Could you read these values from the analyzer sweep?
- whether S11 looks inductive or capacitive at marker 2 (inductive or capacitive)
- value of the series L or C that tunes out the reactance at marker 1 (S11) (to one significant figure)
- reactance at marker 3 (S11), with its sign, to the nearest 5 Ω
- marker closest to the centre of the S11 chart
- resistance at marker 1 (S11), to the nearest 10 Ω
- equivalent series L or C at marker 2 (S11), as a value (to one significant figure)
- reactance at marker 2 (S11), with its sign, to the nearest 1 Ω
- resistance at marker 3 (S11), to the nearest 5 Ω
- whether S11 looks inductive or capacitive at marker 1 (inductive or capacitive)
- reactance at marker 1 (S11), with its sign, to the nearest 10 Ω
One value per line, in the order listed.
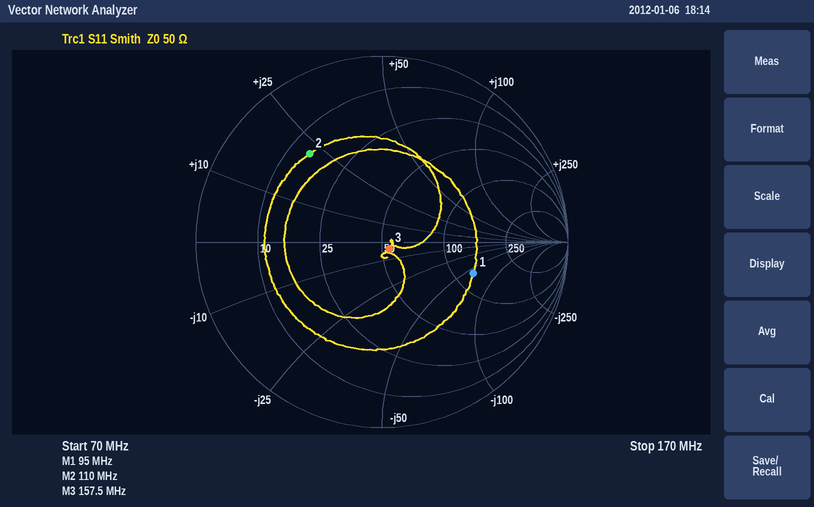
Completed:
inductive
100 nH
-5 Ω
marker 3
130 Ω
30 nH
+22 Ω
55 Ω
capacitive
-60 Ω
